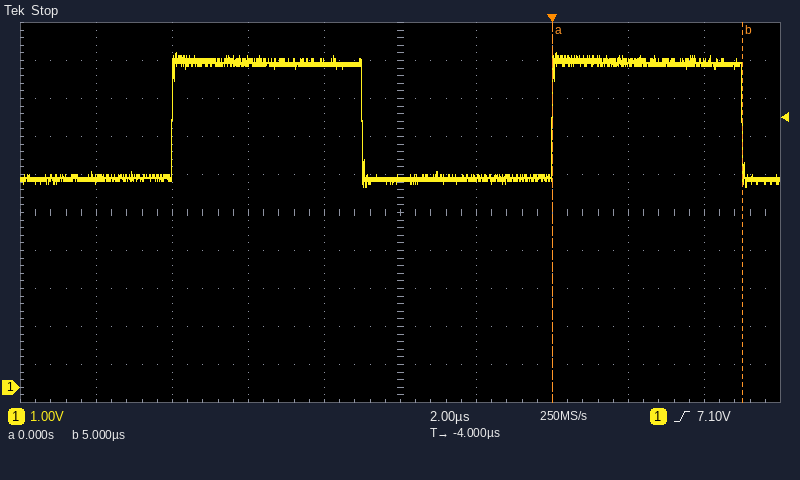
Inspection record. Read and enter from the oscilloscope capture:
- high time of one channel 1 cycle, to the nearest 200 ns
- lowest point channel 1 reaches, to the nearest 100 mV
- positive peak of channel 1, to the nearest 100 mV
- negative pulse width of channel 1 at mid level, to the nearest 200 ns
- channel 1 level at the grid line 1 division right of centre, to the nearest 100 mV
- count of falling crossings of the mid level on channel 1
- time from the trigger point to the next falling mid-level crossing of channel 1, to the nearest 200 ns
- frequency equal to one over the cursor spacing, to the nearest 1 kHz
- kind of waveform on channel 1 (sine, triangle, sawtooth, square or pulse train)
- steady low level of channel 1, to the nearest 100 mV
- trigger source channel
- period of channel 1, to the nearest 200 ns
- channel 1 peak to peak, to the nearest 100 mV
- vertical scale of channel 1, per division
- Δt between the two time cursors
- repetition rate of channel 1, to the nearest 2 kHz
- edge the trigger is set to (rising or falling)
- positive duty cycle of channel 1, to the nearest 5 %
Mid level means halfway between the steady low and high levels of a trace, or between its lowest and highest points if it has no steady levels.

5.0 µs
5.3 V
8.8 V
5.0 µs
5.5 V
2
5.0 µs
200 kHz
square
5.5 V
channel 1
10.0 µs
3.5 V
1 V
5.0 µs
100 kHz
rising
50 %
